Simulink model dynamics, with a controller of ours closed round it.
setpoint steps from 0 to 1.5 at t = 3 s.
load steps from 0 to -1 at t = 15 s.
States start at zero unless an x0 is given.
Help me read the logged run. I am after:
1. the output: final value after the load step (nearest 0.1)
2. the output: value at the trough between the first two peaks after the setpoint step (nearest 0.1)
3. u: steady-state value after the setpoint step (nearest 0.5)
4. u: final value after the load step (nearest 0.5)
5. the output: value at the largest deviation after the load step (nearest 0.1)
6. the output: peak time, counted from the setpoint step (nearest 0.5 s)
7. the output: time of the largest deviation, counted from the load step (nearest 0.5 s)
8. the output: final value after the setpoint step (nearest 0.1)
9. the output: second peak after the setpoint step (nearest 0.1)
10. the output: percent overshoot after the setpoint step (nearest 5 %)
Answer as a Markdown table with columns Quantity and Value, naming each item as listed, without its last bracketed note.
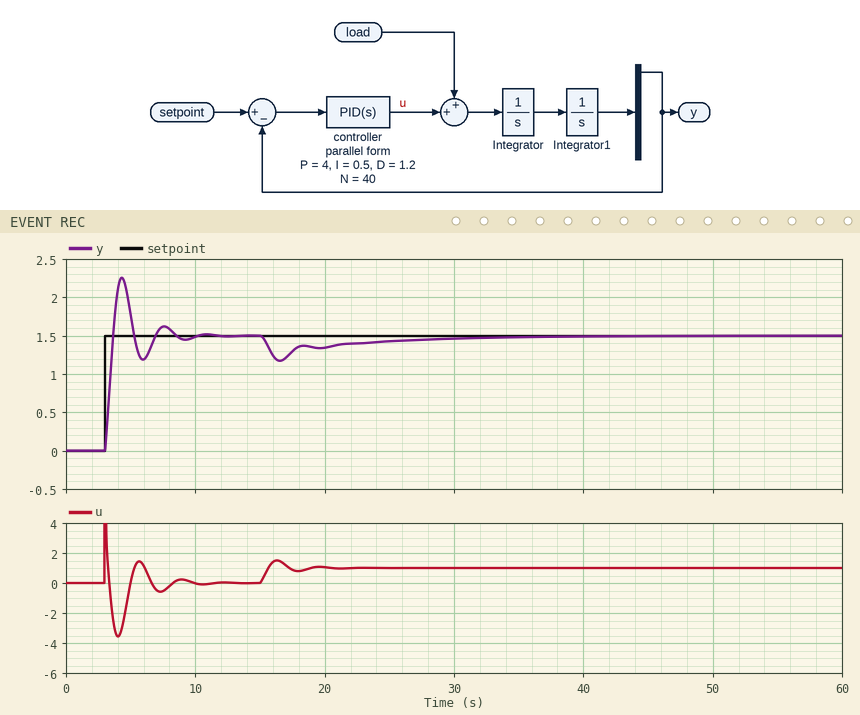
| Quantity | Value |
|---|---|
| the output: final value after the load step | 1.5 |
| the output: value at the trough between the first two peaks after the setpoint step | 1.2 |
| u: steady-state value after the setpoint step | 0.0 |
| u: final value after the load step | 1.0 |
| the output: value at the largest deviation after the load step | 1.2 |
| the output: peak time, counted from the setpoint step | 1.5 s |
| the output: time of the largest deviation, counted from the load step | 1.5 s |
| the output: final value after the setpoint step | 1.5 |
| the output: second peak after the setpoint step | 1.6 |
| the output: percent overshoot after the setpoint step | 50 % |
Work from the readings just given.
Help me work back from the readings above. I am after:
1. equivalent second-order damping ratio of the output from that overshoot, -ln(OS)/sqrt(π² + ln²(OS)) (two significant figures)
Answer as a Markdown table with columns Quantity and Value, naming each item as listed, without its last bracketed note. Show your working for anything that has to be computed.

| Quantity | Value |
|---|---|
| equivalent second-order damping ratio of the output from that overshoot, -ln(OS)/sqrt(π² + ln²(OS)) | ln(0.5) = -0.693; 0.693 / sqrt(9.870 + 0.480) = 0.22 |
